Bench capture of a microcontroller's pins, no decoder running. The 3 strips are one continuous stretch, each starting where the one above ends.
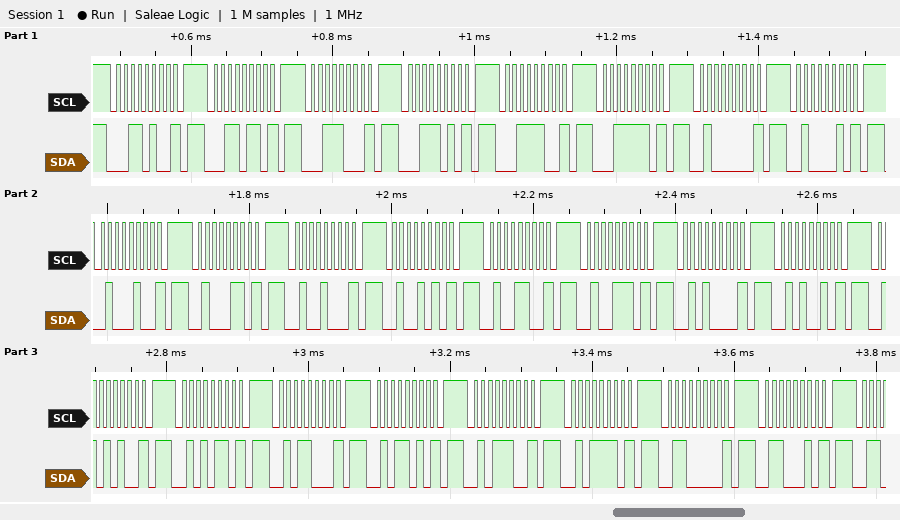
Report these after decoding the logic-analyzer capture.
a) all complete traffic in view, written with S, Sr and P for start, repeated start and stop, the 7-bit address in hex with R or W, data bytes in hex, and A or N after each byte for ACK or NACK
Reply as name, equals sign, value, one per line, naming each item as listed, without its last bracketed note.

all complete traffic in view, written with S, Sr and P for start, repeated start and stop, the 7-bit address in hex with R or W, data bytes in hex, and A or N after each byte for ACK or NACK = S 1AW N P S 1BW N P S 1CW N P S 1DW N P S 1EW N P S 1FW N P S 20W N P S 21W N P S 22W N P S 23W N P S 24W N P S 25W N P S 26W N P S 27W N P S 28W N P S 29W N P S 2AW N P S 2BW N P S 2CW N P S 2DW N P S 2EW N P S 2FW N P S 30W N P S 31W N P
